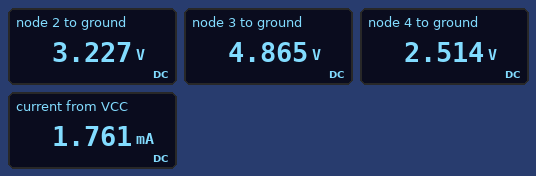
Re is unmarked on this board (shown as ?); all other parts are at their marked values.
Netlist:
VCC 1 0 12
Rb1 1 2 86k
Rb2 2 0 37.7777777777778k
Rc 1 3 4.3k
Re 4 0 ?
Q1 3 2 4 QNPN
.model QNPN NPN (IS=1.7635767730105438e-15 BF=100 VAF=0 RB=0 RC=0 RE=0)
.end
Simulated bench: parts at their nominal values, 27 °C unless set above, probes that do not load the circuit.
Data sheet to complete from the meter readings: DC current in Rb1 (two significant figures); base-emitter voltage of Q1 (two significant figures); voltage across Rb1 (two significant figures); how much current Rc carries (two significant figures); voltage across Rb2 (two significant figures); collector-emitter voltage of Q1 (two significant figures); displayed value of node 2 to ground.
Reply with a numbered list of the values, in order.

1. 100 µA
2. 710 mV
3. 8.8 V
4. 1.7 mA
5. 3.2 V
6. 2.4 V
7. 3.227 V
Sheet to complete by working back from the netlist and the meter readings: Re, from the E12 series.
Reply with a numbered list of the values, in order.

1. 1.5 kΩ
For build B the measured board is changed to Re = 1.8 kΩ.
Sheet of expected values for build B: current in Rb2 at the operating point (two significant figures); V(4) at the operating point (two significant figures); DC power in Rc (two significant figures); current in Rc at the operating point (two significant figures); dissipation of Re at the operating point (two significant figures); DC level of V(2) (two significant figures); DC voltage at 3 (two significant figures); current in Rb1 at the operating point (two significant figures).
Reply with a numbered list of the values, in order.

1. 87 µA
2. 2.6 V
3. 8.7 mW
4. 1.4 mA
5. 3.7 mW
6. 3.3 V
7. 5.9 V
8. 100 µA
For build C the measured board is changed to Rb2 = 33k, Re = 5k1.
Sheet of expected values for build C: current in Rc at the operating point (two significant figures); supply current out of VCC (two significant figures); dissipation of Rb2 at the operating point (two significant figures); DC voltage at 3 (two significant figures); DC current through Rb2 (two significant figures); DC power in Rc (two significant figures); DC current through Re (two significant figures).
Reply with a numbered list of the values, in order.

1. 490 µA
2. 590 µA
3. 310 µW
4. 9.9 V
5. 97 µA
6. 1.0 mW
7. 500 µA
